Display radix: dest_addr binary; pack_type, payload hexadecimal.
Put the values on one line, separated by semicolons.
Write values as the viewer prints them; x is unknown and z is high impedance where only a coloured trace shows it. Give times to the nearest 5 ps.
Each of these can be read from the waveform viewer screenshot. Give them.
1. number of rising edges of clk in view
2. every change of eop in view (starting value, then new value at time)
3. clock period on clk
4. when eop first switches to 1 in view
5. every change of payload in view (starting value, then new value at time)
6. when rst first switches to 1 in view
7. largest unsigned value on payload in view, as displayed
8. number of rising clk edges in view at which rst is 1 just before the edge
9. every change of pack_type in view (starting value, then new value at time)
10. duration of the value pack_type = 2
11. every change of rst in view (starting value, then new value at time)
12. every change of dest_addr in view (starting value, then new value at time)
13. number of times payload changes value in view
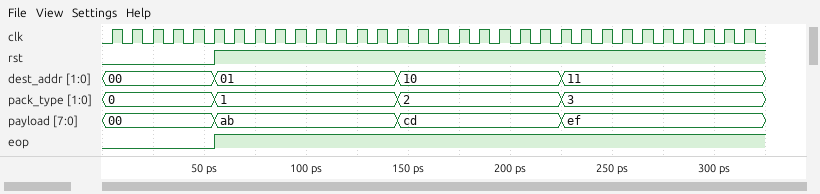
32; 0, 1 at 55 ps; 10 ps; 55 ps; 00, ab at 55 ps, cd at 145 ps, ef at 225 ps; 55 ps; ef; 26; 0, 1 at 55 ps, 2 at 145 ps, 3 at 225 ps; 80 ps; 0, 1 at 55 ps; 00, 01 at 55 ps, 10 at 145 ps, 11 at 225 ps; 3
